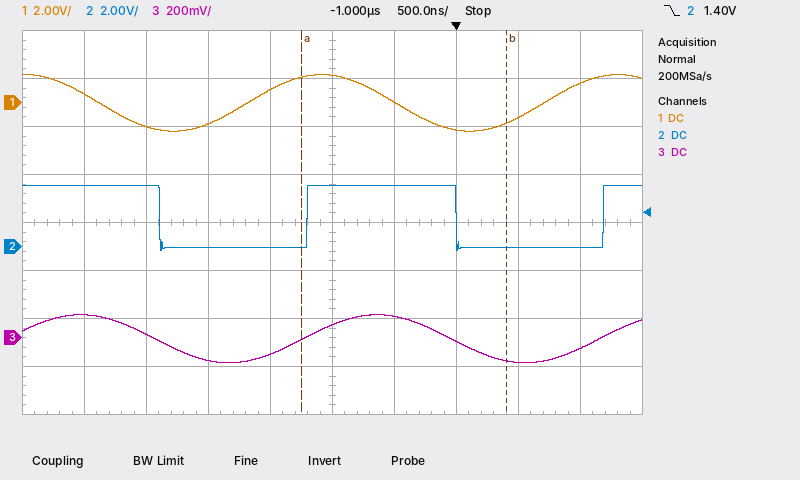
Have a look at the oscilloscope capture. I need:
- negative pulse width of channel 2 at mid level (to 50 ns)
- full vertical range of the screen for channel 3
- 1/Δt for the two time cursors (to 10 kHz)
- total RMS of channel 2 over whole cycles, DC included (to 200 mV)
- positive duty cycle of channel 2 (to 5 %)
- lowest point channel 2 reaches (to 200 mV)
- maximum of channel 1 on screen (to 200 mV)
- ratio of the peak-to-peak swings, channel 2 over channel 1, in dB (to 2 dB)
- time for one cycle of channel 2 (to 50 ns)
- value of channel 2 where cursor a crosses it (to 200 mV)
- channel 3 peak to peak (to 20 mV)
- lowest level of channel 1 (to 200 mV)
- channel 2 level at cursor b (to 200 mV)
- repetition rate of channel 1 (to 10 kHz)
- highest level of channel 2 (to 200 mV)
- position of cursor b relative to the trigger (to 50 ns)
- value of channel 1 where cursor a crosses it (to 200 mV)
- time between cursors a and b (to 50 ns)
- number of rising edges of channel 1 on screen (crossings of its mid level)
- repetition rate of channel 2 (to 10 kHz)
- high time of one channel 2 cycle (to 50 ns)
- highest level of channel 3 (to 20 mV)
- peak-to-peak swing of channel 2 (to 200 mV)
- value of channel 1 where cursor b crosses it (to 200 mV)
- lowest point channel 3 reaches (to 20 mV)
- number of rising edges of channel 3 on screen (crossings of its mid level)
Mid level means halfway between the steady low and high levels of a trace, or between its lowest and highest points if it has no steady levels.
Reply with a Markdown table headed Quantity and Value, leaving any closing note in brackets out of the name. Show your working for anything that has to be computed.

| Quantity | Value |
|---|---|
| negative pulse width of channel 2 at mid level | 1.20 µs |
| full vertical range of the screen for channel 3 | 1.6 V |
| 1/Δt for the two time cursors | 1 / 1.65 µs ≈ 610 kHz |
| total RMS of channel 2 over whole cycles, DC included | √(0.5 × (2.6 V)² + 0.5 × (-200 mV)²) ≈ 1.8 V |
| positive duty cycle of channel 2 | 1.20 µs / 2.40 µs ≈ 50 % |
| lowest point channel 2 reaches | -200 mV |
| maximum of channel 1 on screen | 1.2 V |
| ratio of the peak-to-peak swings, channel 2 over channel 1, in dB | 20 log10(2.8 V / 2.4 V) ≈ 1.34 dB, so 2 dB to the nearest 2 dB |
| time for one cycle of channel 2 | 2.40 µs |
| value of channel 2 where cursor a crosses it | 0.0 V |
| channel 3 peak to peak | 100 mV − (-100 mV) = 200 mV |
| lowest level of channel 1 | -1.2 V |
| channel 2 level at cursor b | 0.0 V |
| repetition rate of channel 1 | 1 / 2.40 µs ≈ 417 kHz, so 420 kHz to the nearest 10 kHz |
| highest level of channel 2 | 2.6 V |
| position of cursor b relative to the trigger | +400 ns |
| value of channel 1 where cursor a crosses it | 1.0 V |
| time between cursors a and b | 1.65 µs |
| number of rising edges of channel 1 on screen | 2 |
| repetition rate of channel 2 | 1 / 2.40 µs ≈ 417 kHz, so 420 kHz to the nearest 10 kHz |
| high time of one channel 2 cycle | 1.20 µs |
| highest level of channel 3 | 100 mV |
| peak-to-peak swing of channel 2 | 2.6 V − (-200 mV) = 2.8 V |
| value of channel 1 where cursor b crosses it | -800 mV |
| lowest point channel 3 reaches | -100 mV |
| number of rising edges of channel 3 on screen | 2 |
